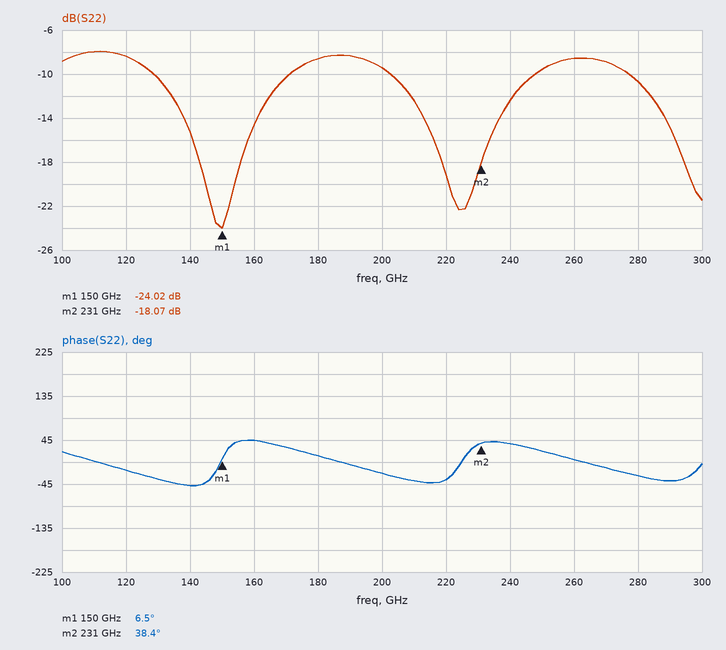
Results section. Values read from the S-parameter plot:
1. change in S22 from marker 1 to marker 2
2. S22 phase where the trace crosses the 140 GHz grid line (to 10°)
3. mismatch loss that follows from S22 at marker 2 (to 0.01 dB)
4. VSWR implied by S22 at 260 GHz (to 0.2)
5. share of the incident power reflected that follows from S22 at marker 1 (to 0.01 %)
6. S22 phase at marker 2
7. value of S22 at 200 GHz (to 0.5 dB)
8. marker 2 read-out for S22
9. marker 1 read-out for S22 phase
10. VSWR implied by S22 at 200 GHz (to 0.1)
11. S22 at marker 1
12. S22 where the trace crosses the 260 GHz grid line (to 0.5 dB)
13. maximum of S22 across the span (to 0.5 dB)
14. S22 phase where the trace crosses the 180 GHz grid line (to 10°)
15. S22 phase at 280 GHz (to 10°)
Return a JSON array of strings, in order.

["5.95 dB", "-50°", "0.07 dB", "2.2", "0.40 %", "38.4°", "-9.5 dB", "-18.07 dB", "6.5°", "2.0", "-24.02 dB", "-8.5 dB", "-8.0 dB", "10°", "-30°"]
